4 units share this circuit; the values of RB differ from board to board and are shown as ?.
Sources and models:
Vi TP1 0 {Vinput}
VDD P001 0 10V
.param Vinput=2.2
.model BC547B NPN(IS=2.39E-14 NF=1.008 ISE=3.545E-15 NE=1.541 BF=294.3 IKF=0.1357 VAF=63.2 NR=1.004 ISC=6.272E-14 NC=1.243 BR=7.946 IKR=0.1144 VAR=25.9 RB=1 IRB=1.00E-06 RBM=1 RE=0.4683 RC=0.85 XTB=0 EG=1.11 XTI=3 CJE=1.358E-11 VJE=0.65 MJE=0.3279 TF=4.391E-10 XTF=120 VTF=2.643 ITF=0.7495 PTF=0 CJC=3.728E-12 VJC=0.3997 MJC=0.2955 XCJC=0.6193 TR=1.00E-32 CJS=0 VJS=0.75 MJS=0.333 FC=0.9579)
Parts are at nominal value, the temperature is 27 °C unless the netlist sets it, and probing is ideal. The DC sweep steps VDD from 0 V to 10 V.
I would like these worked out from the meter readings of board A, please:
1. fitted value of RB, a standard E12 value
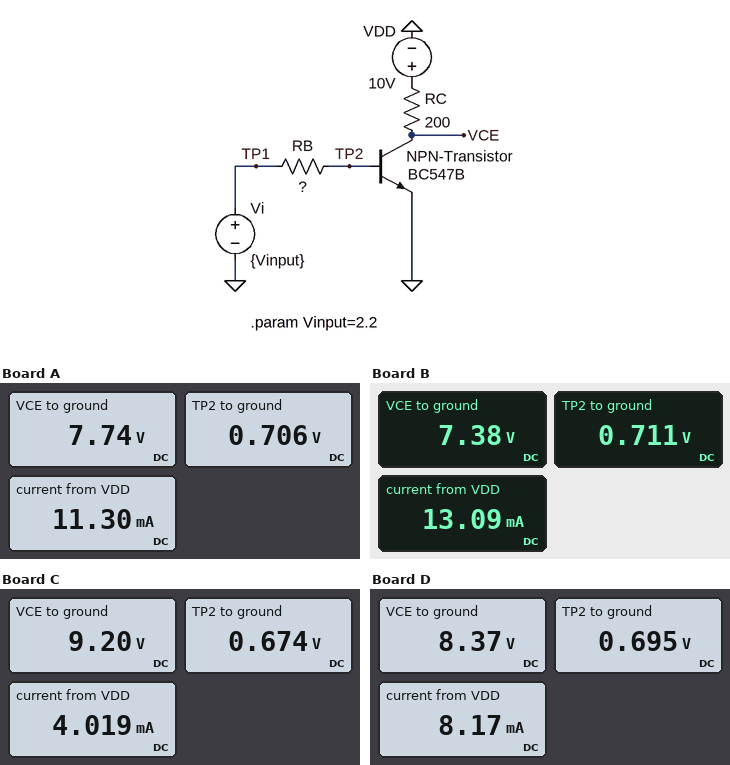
39 kΩ
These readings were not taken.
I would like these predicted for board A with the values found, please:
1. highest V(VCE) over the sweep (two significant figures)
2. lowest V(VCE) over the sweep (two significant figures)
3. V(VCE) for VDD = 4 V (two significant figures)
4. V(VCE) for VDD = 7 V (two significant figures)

7.7 V
4.3 mV
1.9 V
4.8 V
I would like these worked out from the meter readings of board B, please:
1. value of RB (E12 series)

33 kΩ
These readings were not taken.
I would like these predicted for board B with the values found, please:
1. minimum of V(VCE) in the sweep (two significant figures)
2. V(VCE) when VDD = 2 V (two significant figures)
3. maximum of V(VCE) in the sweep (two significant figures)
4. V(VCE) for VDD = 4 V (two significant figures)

4.5 mV
150 mV
7.4 V
1.6 V
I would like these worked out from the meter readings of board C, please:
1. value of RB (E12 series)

120 kΩ
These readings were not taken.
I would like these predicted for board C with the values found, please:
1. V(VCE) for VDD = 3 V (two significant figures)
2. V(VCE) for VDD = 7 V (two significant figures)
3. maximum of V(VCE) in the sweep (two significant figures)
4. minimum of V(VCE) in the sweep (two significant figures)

2.3 V
6.2 V
9.2 V
2.5 mV
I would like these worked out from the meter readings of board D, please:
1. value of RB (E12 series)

56 kΩ
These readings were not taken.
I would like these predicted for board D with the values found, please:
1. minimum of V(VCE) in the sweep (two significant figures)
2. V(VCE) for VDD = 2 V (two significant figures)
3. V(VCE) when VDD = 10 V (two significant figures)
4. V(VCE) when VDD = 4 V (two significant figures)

3.7 mV
550 mV
8.4 V
2.5 V
